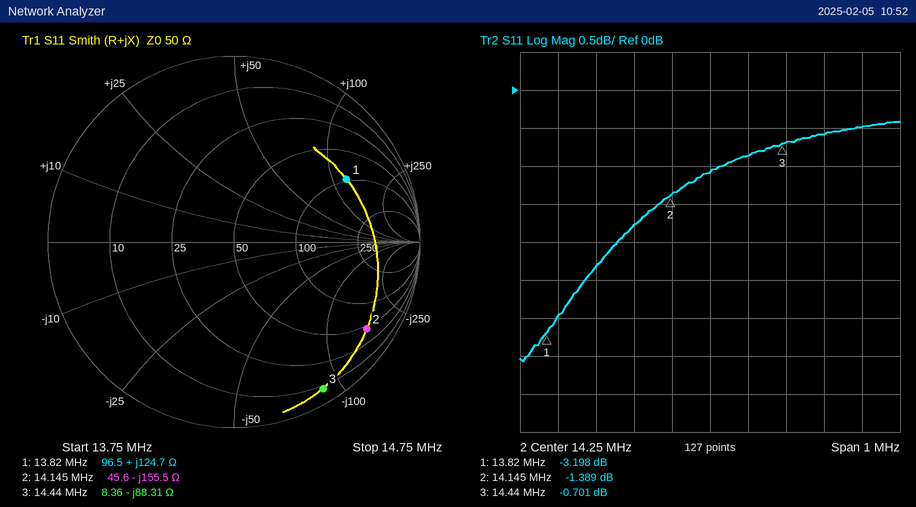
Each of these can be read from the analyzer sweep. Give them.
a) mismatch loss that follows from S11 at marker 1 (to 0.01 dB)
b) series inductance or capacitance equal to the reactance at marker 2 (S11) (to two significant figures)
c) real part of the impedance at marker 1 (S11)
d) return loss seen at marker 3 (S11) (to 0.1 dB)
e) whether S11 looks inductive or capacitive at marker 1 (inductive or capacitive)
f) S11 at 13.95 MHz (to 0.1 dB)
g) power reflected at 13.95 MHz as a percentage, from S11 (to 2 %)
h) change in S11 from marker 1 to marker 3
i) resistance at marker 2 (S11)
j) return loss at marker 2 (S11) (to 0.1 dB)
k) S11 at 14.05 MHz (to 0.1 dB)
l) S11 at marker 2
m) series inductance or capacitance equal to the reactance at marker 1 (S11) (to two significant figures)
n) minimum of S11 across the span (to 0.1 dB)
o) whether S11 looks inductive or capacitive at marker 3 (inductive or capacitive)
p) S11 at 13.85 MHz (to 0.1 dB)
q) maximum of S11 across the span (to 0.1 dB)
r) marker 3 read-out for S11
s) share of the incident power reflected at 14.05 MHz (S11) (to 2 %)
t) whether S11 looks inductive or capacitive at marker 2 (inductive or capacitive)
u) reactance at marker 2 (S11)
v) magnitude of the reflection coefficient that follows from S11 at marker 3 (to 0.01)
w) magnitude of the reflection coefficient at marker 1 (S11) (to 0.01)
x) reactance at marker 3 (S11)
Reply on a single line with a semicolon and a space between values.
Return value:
2.83 dB; 72 pF; 96.5 Ω; 0.7 dB; inductive; -2.3 dB; 58 %; 2.497 dB; 45.6 Ω; 1.4 dB; -1.8 dB; -1.389 dB; 1.4 µH; -3.6 dB; capacitive; -3.0 dB; -0.4 dB; -0.701 dB; 66 %; capacitive; -155.5 Ω; 0.92; 0.69; -88.31 Ω
